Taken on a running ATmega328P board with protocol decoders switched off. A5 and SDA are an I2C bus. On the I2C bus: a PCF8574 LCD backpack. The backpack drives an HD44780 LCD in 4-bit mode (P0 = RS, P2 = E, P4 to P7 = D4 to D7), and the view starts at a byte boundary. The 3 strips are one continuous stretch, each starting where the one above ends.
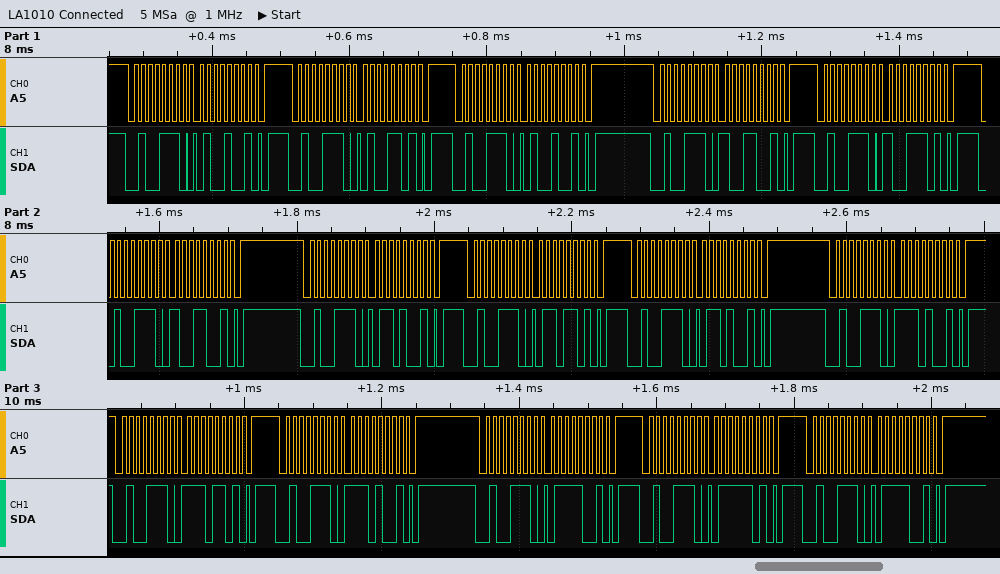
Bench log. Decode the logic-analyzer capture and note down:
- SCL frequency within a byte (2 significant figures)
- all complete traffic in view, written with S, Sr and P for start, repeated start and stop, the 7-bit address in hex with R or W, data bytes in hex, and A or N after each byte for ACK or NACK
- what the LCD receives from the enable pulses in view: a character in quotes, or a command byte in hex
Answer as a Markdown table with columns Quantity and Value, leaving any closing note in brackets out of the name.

| Quantity | Value |
|---|---|
| SCL frequency within a byte | 100 kHz |
| all complete traffic in view, written with S, Sr and P for start, repeated start and stop, the 7-bit address in hex with R or W, data bytes in hex, and A or N after each byte for ACK or NACK | S 27W A 49 A P S 27W A 4D A P S 27W A 49 A P S 27W A 99 A P S 27W A 9D A P S 27W A 99 A P S 27W A 69 A P S 27W A 6D A P S 27W A 69 A P S 27W A E9 A P S 27W A ED A P S 27W A E9 A P S 27W A 79 A P S 27W A 7D A P S 27W A 79 A P |
| what the LCD receives from the enable pulses in view: a character in quotes, or a command byte in hex | 'I' 'n' |
